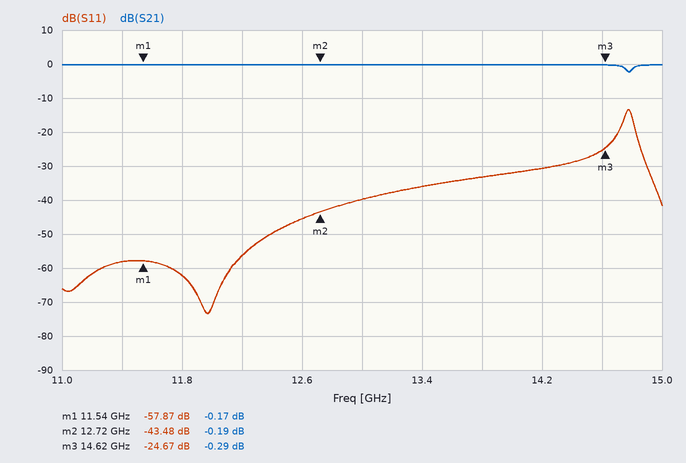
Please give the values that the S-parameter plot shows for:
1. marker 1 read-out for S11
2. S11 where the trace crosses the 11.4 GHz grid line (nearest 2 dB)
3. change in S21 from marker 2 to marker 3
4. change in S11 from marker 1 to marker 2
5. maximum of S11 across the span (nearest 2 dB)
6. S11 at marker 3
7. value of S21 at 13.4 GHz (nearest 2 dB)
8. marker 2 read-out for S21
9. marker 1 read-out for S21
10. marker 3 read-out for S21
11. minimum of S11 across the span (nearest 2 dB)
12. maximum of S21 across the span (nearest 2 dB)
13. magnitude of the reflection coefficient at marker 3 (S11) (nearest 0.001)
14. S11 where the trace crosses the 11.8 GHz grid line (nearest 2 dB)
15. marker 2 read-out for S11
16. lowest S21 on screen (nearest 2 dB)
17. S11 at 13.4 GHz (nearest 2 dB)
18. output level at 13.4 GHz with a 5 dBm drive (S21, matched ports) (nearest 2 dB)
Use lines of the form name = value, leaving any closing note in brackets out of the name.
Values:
marker 1 read-out for S11 = -57.87 dB
S11 where the trace crosses the 11.4 GHz grid line = -58 dB
change in S21 from marker 2 to marker 3 = -0.10 dB
change in S11 from marker 1 to marker 2 = 14.39 dB
maximum of S11 across the span = -14 dB
S11 at marker 3 = -24.67 dB
value of S21 at 13.4 GHz = 0 dB
marker 2 read-out for S21 = -0.19 dB
marker 1 read-out for S21 = -0.17 dB
marker 3 read-out for S21 = -0.29 dB
minimum of S11 across the span = -74 dB
maximum of S21 across the span = 0 dB
magnitude of the reflection coefficient at marker 3 (S11) = 0.058
S11 where the trace crosses the 11.8 GHz grid line = -62 dB
marker 2 read-out for S11 = -43.48 dB
lowest S21 on screen = -2 dB
S11 at 13.4 GHz = -36 dB
output level at 13.4 GHz with a 5 dBm drive (S21, matched ports) = 4 dBm
